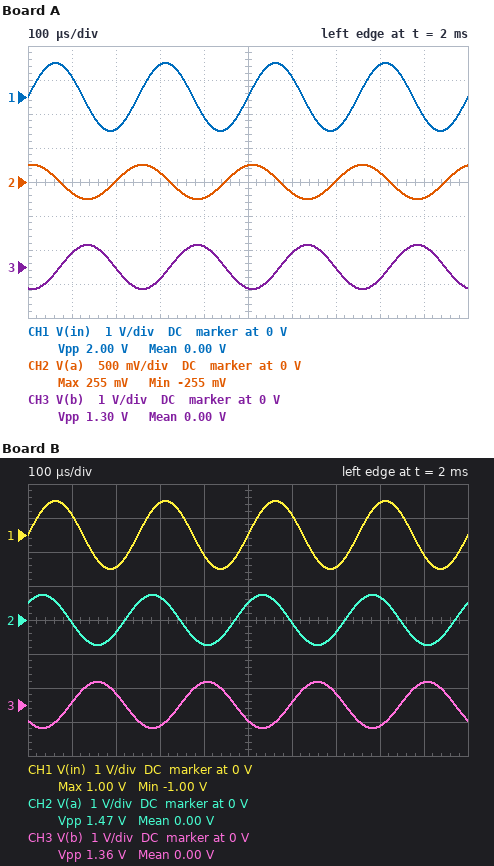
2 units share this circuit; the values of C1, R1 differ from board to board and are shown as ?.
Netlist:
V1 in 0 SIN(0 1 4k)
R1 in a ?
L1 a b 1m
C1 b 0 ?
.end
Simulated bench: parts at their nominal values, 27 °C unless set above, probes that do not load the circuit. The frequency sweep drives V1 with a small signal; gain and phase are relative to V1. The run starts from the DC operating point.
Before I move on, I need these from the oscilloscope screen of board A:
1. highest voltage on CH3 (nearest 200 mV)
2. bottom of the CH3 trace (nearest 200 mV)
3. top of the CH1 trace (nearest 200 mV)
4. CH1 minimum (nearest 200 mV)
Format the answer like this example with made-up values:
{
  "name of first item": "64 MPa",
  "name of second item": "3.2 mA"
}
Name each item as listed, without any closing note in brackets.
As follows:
{
  "highest voltage on CH3": "600 mV",
  "bottom of the CH3 trace": "-600 mV",
  "top of the CH1 trace": "1.0 V",
  "CH1 minimum": "-1.0 V"
}
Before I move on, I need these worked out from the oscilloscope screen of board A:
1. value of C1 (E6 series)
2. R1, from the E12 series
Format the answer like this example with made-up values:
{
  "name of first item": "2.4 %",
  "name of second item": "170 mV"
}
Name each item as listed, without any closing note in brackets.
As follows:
{
  "value of C1": "2.2 µF",
  "R1, from the E12 series": "27 Ω"
}
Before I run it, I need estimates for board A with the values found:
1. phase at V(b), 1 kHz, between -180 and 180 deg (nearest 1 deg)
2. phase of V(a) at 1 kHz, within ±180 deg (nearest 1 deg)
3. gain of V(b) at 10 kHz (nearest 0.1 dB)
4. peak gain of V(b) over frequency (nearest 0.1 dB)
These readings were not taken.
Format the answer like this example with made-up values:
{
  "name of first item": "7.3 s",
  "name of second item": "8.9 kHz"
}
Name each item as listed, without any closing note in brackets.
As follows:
{
  "phase at V(b), 1 kHz, between -180 and 180 deg": "-22 deg",
  "phase of V(a) at 1 kHz, within ±180 deg": "-22 deg",
  "gain of V(b) at 10 kHz": "-18.6 dB",
  "peak gain of V(b) over frequency": "0.2 dB"
}
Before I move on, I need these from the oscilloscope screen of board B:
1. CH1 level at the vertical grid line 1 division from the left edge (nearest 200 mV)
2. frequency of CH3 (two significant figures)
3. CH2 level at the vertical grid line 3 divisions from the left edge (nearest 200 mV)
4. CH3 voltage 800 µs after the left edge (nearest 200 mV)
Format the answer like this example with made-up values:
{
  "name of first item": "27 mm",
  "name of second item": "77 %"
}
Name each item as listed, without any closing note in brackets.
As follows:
{
  "CH1 level at the vertical grid line 1 division from the left edge": "600 mV",
  "frequency of CH3": "4.0 kHz",
  "CH2 level at the vertical grid line 3 divisions from the left edge": "600 mV",
  "CH3 voltage 800 µs after the left edge": "-600 mV"
}
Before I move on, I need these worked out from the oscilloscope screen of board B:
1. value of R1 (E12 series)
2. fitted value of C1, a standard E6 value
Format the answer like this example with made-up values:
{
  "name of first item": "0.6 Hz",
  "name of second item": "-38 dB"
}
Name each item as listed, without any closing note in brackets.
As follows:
{
  "value of R1": "12 Ω",
  "fitted value of C1, a standard E6 value": "3.3 µF"
}
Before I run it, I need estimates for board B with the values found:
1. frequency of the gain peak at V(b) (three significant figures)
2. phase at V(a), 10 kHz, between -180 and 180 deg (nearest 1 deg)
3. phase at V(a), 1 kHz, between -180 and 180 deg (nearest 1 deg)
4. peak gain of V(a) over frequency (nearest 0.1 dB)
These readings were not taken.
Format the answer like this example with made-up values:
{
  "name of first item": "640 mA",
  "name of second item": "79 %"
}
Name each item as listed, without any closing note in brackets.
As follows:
{
  "frequency of the gain peak at V(b)": "2.42 kHz",
  "phase at V(a), 10 kHz, between -180 and 180 deg": "12 deg",
  "phase at V(a), 1 kHz, between -180 and 180 deg": "-16 deg",
  "peak gain of V(a) over frequency": "0 dB"
}
